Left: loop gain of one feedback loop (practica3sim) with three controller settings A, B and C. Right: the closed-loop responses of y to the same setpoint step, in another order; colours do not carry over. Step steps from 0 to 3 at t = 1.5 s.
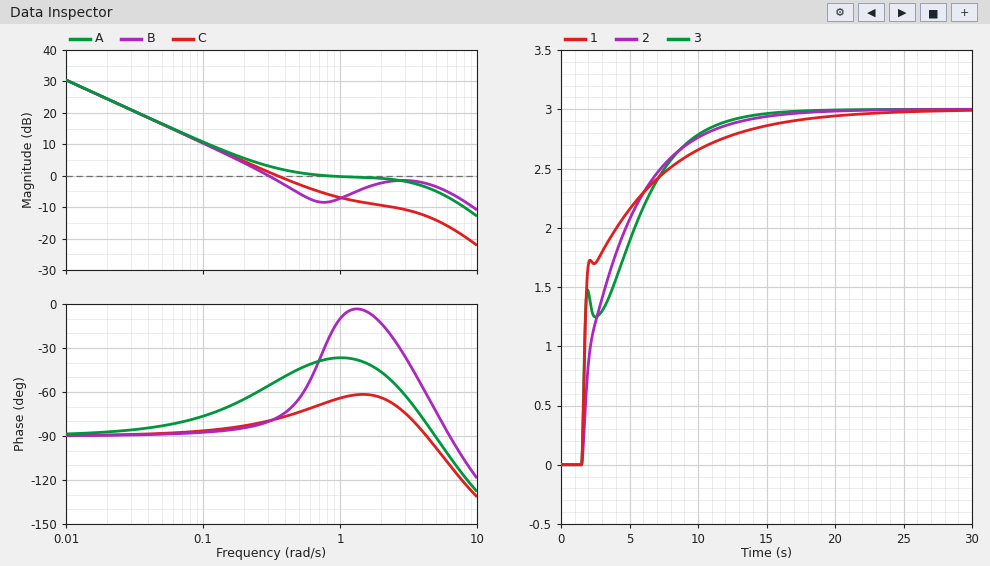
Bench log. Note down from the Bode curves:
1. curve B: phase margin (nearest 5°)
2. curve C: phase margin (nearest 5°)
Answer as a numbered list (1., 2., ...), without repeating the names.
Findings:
1. 100°
2. 100°
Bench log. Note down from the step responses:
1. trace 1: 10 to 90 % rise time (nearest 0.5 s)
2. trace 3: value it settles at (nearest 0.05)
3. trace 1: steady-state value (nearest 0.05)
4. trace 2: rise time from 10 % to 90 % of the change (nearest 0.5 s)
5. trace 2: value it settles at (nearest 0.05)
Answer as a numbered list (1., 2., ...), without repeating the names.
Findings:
1. 9.0 s
2. 3.00
3. 3.00
4. 7.5 s
5. 3.00
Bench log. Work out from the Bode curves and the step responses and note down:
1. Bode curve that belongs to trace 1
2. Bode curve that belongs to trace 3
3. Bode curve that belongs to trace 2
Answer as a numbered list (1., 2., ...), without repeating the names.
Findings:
1. A
2. B
3. C
